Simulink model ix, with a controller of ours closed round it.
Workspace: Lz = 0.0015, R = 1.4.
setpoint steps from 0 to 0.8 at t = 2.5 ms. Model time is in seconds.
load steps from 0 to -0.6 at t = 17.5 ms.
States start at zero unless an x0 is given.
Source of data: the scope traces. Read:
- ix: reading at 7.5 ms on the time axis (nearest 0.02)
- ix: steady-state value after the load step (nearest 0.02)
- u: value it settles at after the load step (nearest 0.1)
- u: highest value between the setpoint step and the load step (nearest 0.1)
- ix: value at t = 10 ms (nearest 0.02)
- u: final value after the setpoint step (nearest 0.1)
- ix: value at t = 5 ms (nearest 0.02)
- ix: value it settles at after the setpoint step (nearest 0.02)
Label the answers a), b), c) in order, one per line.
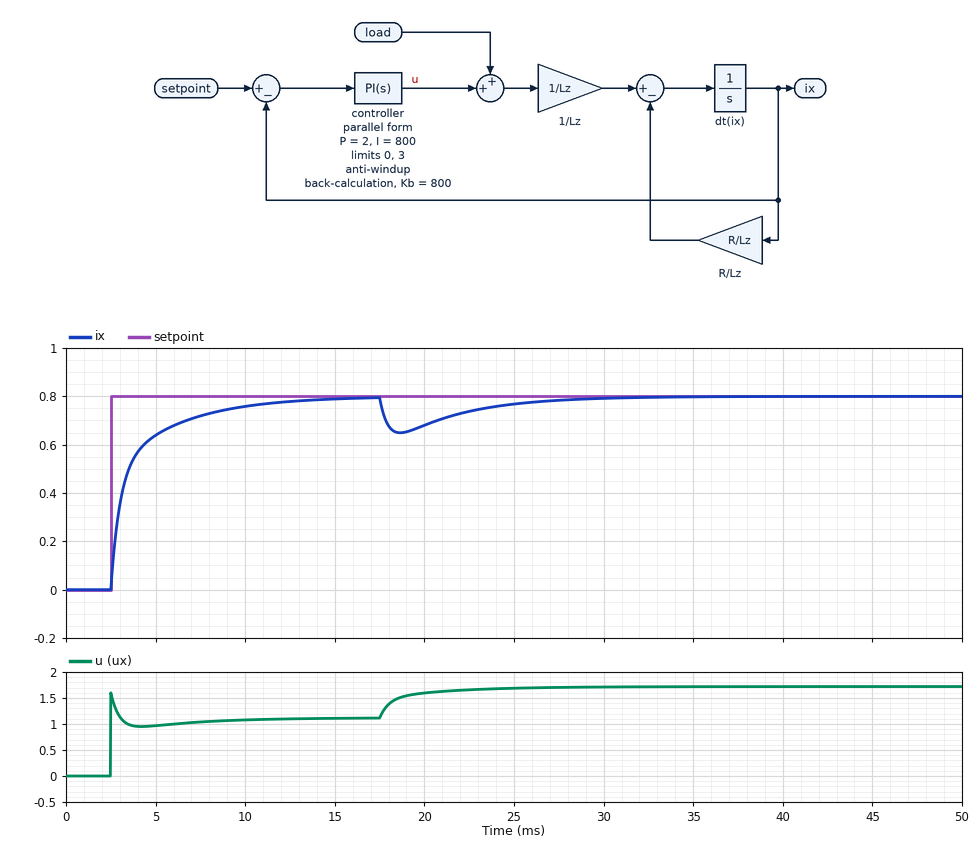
a) 0.72
b) 0.80
c) 1.7
d) 1.6
e) 0.76
f) 1.1
g) 0.64
h) 0.80
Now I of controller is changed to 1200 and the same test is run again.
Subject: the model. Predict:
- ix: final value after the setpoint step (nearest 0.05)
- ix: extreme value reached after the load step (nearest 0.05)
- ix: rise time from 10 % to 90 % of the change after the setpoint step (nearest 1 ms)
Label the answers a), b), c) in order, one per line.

a) 0.80
b) 0.65
c) 3 ms
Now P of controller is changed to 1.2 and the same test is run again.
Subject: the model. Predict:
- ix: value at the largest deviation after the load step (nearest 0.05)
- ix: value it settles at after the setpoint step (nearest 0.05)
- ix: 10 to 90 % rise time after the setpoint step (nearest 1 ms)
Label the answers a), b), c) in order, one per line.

a) 0.60
b) 0.80
c) 4 ms
